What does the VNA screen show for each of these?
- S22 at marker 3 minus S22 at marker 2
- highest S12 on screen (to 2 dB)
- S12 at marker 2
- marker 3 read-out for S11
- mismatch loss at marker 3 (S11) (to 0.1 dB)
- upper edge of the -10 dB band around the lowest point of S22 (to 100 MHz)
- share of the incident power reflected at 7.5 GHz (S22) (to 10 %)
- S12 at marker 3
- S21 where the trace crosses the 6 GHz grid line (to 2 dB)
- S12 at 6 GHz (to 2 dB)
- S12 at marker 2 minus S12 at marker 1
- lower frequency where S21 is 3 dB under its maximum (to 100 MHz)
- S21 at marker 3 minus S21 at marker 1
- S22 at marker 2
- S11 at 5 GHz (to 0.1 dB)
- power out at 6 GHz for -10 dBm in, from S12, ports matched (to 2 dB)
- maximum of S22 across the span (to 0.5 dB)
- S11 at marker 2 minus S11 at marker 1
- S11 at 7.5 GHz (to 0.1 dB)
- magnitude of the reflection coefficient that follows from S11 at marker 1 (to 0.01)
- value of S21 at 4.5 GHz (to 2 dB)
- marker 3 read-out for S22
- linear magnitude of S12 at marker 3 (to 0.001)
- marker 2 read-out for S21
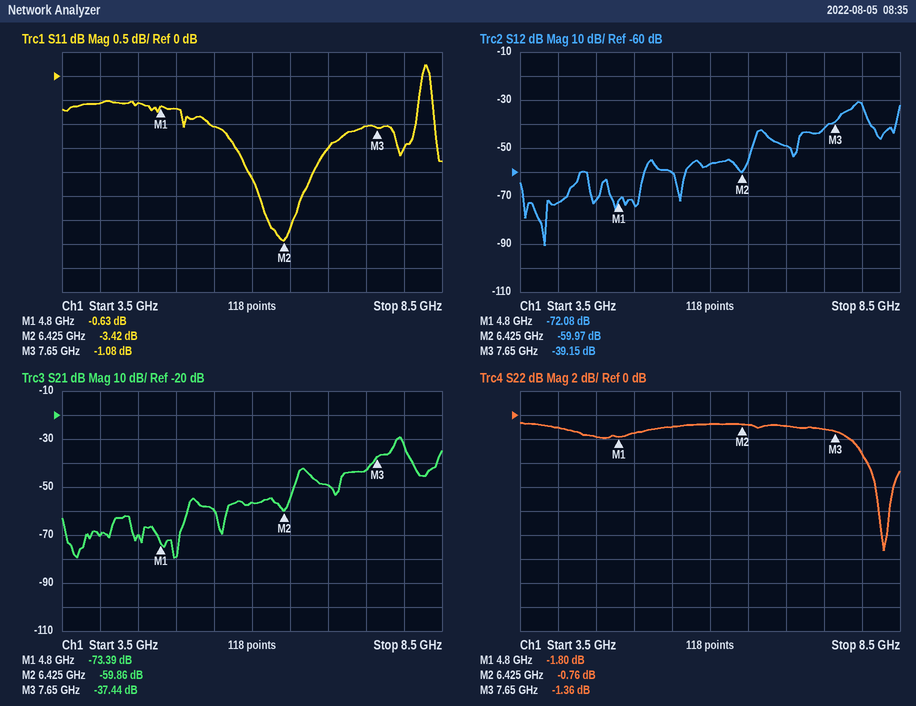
-0.60 dB
-30 dB
-59.97 dB
-1.08 dB
6.6 dB
8.3 GHz
80 %
-39.15 dB
-56 dB
-56 dB
12.11 dB
7.9 GHz
35.95 dB
-0.76 dB
-0.7 dB
-66 dBm
-0.5 dB
-2.79 dB
-1.0 dB
0.93
-70 dB
-1.36 dB
0.011
-59.86 dB
